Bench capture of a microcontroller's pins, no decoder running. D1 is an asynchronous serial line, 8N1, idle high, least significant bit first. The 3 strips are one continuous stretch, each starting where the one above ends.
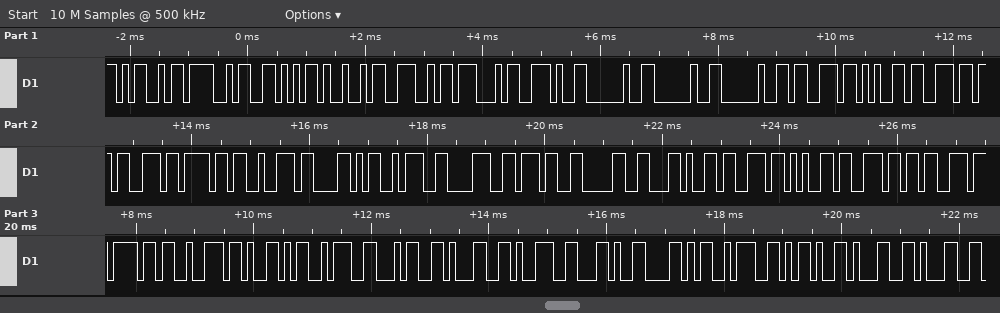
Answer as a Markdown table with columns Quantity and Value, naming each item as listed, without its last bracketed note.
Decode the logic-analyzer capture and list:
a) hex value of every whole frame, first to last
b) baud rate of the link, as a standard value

| Quantity | Value |
|---|---|
| hex value of every whole frame, first to last | 0x4D 0x4F 0x56 0x49 0x4E 0x47 0x2E 0x20 0x20 0x20 0x73 0x65 0x6E 0x73 0x6F 0x72 0x58 0x3A 0x38 0x37 0x30 0x2C 0x73 0x65 0x6E 0x73 0x6F 0x72 0x59 0x3A 0x34 0x31 0x39 0x2C 0x58 0x3A 0x2D 0x31 0x31 |
| baud rate of the link, as a standard value | 9600 baud |
